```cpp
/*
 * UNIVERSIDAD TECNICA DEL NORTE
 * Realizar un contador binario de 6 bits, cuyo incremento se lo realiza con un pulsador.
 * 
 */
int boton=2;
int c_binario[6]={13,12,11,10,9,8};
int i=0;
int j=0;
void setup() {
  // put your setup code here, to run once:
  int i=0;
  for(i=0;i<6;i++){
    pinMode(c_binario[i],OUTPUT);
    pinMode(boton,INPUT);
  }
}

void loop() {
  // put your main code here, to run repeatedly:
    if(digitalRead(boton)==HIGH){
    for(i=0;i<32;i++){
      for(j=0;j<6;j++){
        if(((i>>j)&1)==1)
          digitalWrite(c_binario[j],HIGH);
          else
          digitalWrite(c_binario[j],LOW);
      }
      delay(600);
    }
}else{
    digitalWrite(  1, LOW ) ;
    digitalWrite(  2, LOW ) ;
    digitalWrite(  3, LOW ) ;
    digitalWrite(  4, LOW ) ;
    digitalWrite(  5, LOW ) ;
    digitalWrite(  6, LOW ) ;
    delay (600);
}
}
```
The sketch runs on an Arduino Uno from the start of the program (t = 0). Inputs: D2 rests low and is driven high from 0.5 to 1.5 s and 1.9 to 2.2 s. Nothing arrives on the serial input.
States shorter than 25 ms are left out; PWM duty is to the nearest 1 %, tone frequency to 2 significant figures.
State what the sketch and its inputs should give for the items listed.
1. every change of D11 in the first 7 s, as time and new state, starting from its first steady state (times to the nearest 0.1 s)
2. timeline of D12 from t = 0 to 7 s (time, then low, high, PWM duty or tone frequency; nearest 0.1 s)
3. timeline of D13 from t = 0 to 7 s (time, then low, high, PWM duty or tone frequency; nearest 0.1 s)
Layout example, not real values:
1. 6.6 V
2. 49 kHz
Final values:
1. 0 s low; 3 s high; 5.4 s low
2. 0 s low; 1.8 s high; 3 s low; 4.2 s high; 5.4 s low; 6.6 s high
3. 0 s low; 1.2 s high; 1.8 s low; 2.4 s high; 3 s low; 3.6 s high; 4.2 s low; 4.8 s high; 5.4 s low; 6 s high; 6.6 s low
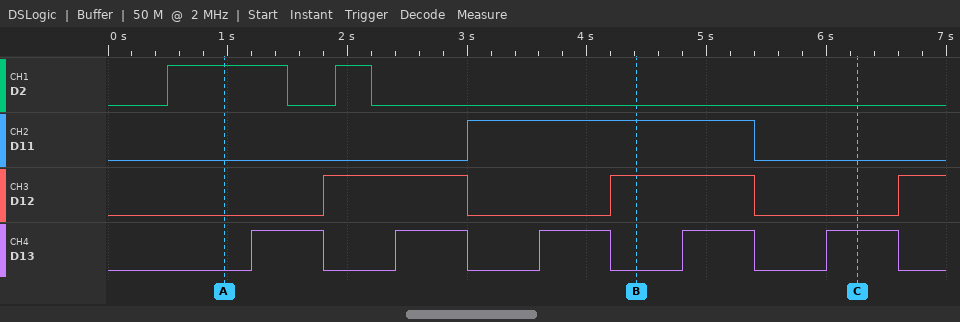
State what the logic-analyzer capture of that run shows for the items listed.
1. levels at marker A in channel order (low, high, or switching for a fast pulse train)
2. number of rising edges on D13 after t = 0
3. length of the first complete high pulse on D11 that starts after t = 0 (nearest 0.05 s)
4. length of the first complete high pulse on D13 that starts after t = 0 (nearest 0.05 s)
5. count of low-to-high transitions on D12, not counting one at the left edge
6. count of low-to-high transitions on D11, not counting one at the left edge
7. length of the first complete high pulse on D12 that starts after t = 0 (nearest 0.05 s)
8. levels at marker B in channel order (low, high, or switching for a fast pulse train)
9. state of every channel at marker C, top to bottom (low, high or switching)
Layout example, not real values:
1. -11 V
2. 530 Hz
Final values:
1. D2 high, D11 low, D12 low, D13 low
2. 5
3. 2.40 s
4. 0.60 s
5. 3
6. 1
7. 1.20 s
8. D2 low, D11 high, D12 high, D13 low
9. D2 low, D11 low, D12 low, D13 high
